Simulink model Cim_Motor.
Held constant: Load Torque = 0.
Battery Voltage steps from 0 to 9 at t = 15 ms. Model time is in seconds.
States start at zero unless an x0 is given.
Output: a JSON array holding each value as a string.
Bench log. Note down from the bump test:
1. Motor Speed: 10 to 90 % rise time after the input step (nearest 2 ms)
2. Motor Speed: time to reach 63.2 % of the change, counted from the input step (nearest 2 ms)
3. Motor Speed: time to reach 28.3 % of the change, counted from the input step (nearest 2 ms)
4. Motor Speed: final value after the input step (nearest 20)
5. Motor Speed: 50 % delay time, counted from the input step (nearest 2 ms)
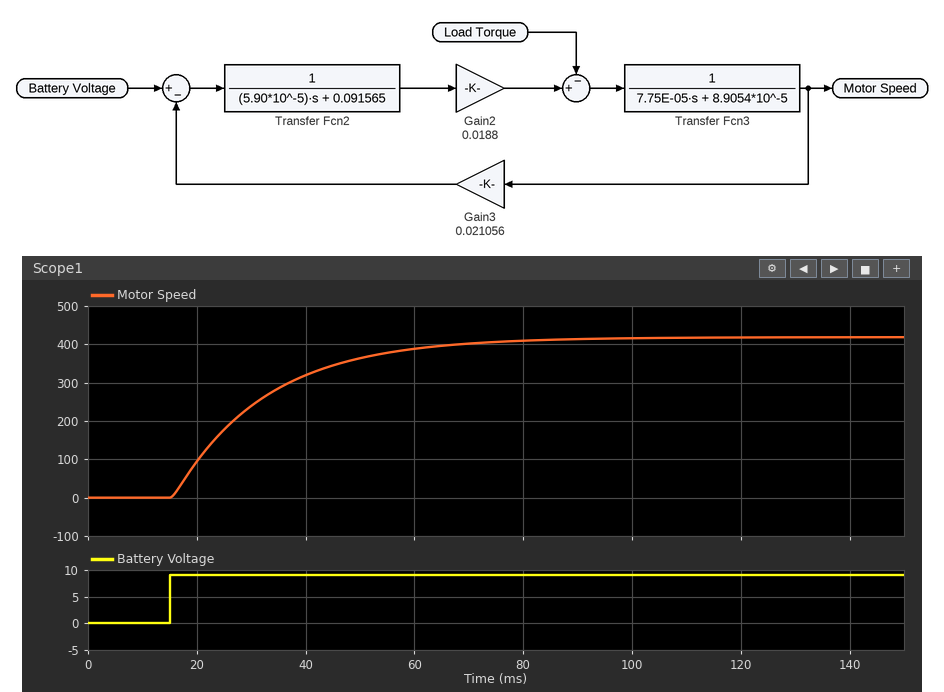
["38 ms", "18 ms", "6 ms", "420", "12 ms"]
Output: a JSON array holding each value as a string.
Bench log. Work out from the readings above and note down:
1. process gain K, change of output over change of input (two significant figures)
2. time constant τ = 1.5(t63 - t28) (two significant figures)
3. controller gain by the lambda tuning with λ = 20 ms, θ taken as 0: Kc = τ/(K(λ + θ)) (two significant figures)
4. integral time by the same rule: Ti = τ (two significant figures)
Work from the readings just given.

["47", "18 ms", "0.019", "18 ms"]
